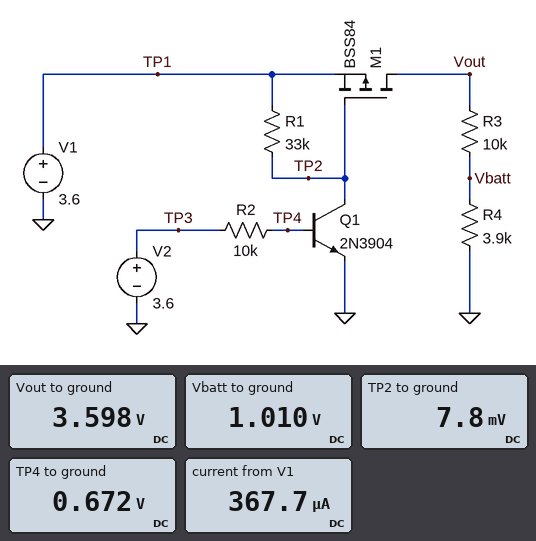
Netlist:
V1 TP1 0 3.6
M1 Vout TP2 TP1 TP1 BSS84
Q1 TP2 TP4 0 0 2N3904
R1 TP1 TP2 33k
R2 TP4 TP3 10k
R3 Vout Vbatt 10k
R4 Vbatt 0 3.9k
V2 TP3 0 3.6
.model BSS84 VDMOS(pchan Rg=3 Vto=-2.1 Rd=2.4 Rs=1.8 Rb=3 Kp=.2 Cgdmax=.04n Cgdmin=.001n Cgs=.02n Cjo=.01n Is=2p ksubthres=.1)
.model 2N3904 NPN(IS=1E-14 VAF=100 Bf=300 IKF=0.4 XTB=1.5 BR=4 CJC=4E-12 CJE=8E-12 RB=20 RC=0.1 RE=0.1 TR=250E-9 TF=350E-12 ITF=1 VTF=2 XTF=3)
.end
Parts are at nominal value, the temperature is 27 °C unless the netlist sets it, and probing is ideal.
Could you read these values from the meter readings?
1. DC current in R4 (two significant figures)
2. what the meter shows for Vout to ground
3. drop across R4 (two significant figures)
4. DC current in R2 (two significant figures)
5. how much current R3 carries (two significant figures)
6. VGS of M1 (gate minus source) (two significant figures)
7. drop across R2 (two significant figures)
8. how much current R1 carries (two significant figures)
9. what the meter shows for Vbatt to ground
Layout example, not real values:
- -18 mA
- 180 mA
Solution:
- 260 µA
- 3.598 V
- 1.0 V
- 290 µA
- 260 µA
- -3.6 V
- 2.9 V
- 110 µA
- 1.010 V
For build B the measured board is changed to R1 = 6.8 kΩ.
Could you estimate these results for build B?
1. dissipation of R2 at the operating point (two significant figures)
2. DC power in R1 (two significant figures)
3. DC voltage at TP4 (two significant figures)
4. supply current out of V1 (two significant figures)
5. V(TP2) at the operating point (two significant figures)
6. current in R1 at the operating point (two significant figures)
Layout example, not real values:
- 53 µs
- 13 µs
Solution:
- 850 µW
- 1.9 mW
- 680 mV
- 790 µA
- 14 mV
- 530 µA
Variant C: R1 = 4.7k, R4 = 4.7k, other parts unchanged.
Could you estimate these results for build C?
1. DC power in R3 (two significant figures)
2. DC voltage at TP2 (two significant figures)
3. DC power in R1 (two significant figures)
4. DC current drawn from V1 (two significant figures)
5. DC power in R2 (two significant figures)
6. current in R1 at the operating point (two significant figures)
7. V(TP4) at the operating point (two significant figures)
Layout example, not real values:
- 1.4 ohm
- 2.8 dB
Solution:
- 600 µW
- 17 mV
- 2.7 mW
- 1.0 mA
- 850 µW
- 760 µA
- 680 mV
